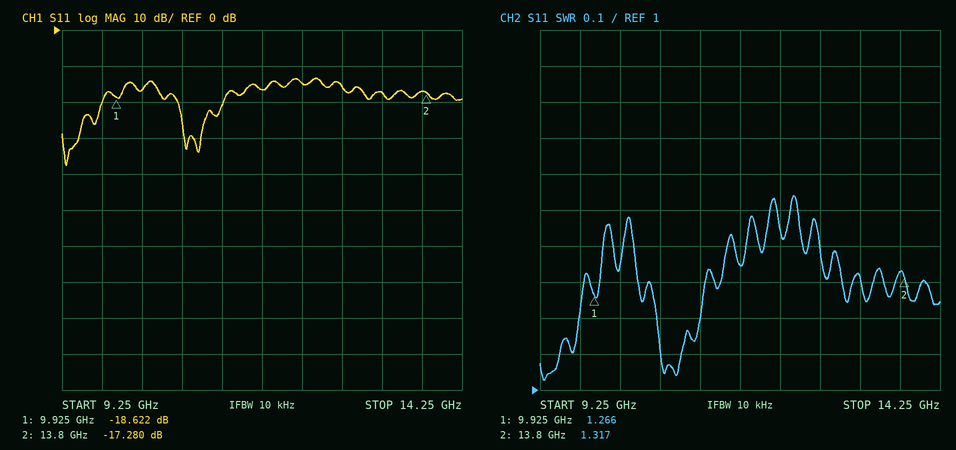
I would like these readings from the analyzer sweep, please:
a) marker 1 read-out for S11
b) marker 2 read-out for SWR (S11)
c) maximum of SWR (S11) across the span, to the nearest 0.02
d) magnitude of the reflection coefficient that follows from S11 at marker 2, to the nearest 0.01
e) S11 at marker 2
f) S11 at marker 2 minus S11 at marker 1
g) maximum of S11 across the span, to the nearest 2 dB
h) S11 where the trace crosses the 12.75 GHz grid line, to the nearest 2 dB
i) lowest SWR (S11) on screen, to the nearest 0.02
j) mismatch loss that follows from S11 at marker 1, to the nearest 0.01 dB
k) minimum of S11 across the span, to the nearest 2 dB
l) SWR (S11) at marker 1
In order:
-18.622 dB
1.317
1.54
0.14
-17.280 dB
1.342 dB
-14 dB
-16 dB
1.02
0.06 dB
-38 dB
1.266
